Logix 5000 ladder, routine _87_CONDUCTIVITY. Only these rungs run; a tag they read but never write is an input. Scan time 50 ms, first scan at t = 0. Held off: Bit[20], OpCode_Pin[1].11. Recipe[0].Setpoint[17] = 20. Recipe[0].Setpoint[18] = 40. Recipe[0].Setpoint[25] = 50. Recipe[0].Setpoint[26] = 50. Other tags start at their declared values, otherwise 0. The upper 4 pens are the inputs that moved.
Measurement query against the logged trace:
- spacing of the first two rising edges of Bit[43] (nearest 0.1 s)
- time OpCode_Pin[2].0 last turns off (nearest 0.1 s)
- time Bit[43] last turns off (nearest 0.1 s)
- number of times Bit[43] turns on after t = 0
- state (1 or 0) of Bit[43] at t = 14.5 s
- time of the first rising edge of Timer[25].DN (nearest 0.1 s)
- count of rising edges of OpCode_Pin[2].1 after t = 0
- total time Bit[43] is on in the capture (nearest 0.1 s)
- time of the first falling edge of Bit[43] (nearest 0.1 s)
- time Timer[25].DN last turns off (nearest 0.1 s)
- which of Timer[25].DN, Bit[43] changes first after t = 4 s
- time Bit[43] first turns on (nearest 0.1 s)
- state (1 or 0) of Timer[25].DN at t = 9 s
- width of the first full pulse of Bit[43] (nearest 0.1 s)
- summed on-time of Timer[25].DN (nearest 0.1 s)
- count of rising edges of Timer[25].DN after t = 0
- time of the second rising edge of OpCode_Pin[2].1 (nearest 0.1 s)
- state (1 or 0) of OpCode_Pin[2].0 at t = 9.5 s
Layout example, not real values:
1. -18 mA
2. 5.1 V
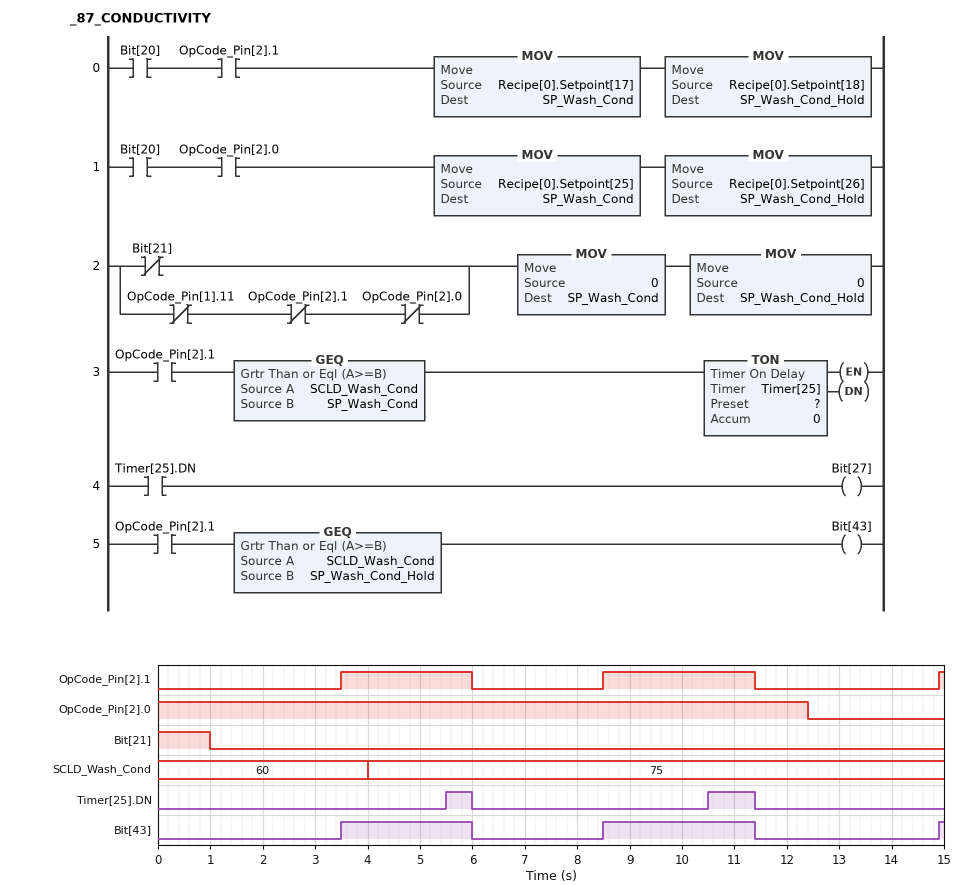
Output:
1. 5.0 s
2. 12.4 s
3. 11.4 s
4. 3
5. 0
6. 5.5 s
7. 3
8. 5.5 s
9. 6.0 s
10. 11.4 s
11. Timer[25].DN
12. 3.5 s
13. 0
14. 2.5 s
15. 1.4 s
16. 2
17. 8.5 s
18. 1
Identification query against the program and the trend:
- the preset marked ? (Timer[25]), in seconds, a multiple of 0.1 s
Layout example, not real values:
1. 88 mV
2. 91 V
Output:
1. 2.0 s
